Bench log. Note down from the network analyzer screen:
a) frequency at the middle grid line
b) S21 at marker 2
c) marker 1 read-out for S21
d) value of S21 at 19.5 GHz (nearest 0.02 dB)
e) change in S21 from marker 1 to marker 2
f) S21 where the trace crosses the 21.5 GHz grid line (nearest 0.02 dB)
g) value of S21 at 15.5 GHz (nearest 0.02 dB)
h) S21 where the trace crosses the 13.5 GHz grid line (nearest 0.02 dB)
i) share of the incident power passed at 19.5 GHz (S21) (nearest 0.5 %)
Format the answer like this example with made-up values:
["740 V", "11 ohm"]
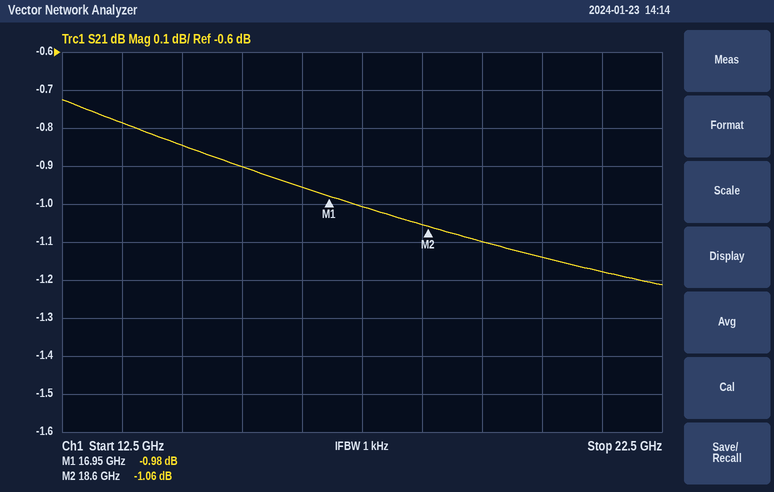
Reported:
["17.5 GHz", "-1.06 dB", "-0.98 dB", "-1.10 dB", "-0.08 dB", "-1.18 dB", "-0.90 dB", "-0.78 dB", "77.5 %"]
